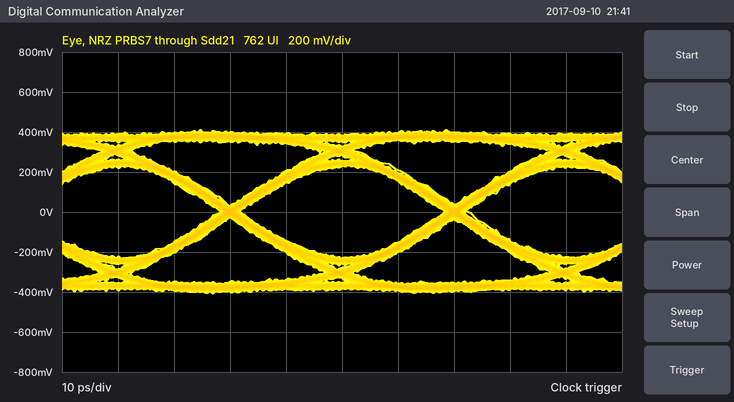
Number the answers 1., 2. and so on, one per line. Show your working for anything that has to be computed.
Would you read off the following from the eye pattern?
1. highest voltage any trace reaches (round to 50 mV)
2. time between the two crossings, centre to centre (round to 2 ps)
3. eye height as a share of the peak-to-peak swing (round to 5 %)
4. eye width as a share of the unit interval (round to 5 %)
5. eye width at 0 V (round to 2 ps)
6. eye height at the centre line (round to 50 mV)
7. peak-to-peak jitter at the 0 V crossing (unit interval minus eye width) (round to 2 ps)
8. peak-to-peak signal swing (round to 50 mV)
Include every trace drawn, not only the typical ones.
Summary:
1. 400 mV
2. 40 ps
3. 450 mV / 800 mV ≈ 56.2 %, so 55 % to the nearest 5 %
4. 36 ps / 40 ps ≈ 90 %
5. 36 ps
6. 450 mV
7. 4 ps
8. 800 mV
